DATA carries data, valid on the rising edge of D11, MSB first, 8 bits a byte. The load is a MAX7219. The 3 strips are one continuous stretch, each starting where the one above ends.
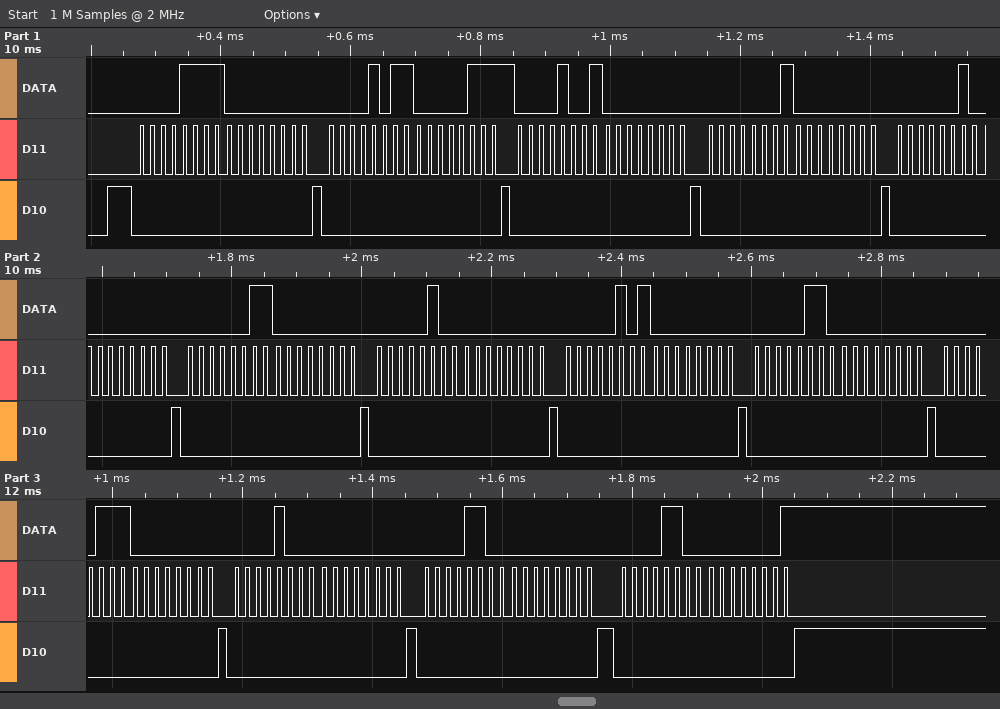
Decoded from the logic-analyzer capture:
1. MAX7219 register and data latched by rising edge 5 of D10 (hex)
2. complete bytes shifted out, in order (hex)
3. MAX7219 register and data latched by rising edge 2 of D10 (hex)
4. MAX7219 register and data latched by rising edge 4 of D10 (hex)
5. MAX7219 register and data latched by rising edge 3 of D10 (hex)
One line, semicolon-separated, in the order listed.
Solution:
register 0x1, data 0x00; 0x0F 0x00 0x0B 0x07 0x09 0x00 0x01 0x00 0x02 0x00 0x03 0x00 0x04 0x00 0x05 0x00 0x06 0x00 0x07 0x00 0x08 0x00 0x0C 0x00 0x0C 0x01; register 0xF, data 0x00; register 0x9, data 0x00; register 0xB, data 0x07
